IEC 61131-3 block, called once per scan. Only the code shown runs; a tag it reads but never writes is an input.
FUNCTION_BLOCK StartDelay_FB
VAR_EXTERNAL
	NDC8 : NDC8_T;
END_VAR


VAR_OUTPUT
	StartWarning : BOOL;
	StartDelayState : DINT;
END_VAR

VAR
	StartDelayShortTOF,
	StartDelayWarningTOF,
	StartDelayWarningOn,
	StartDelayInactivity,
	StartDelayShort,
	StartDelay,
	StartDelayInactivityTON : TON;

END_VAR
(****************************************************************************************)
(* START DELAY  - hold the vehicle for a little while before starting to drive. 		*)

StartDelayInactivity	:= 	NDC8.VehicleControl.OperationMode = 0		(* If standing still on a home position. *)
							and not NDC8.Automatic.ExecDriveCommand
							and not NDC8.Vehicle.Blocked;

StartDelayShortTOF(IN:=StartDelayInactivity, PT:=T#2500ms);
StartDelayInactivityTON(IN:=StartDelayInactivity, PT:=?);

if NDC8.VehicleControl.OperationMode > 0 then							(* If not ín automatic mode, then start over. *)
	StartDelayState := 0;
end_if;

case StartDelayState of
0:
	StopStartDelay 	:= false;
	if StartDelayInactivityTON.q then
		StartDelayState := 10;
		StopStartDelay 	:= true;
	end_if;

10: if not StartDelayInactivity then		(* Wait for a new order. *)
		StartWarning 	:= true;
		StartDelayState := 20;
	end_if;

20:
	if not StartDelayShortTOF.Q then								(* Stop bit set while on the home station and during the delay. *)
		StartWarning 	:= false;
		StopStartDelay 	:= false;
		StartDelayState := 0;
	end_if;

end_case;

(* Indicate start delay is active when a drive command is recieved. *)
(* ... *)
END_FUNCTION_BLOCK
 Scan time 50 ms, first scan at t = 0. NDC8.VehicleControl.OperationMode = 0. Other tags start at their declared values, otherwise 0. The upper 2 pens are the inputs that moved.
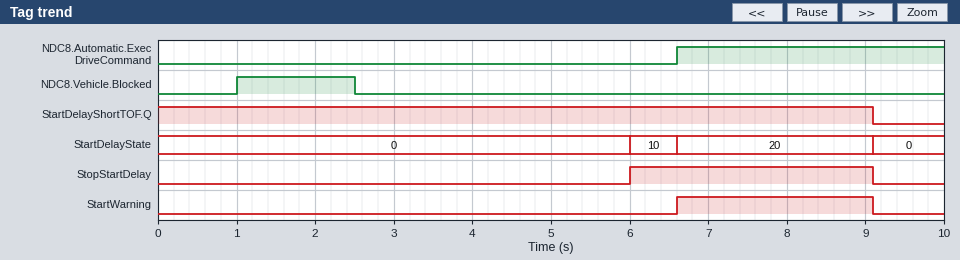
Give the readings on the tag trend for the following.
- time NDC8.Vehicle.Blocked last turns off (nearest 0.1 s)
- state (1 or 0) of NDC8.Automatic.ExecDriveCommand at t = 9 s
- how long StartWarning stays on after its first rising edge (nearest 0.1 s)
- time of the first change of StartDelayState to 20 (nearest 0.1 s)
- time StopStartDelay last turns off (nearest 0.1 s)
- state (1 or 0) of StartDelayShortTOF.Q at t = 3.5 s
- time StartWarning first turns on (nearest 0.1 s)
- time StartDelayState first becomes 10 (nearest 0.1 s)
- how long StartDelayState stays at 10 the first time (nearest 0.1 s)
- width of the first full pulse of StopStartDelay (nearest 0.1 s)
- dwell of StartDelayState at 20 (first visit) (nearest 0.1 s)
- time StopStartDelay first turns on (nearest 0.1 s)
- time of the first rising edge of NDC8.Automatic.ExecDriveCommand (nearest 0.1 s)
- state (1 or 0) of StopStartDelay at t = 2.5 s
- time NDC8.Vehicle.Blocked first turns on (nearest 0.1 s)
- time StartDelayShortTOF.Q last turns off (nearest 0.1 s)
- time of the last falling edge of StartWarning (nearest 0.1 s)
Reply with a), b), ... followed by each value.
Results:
a) 2.5 s
b) 1
c) 2.5 s
d) 6.6 s
e) 9.1 s
f) 1
g) 6.6 s
h) 6.0 s
i) 0.6 s
j) 3.1 s
k) 2.5 s
l) 6.0 s
m) 6.6 s
n) 0
o) 1.0 s
p) 9.1 s
q) 9.1 s
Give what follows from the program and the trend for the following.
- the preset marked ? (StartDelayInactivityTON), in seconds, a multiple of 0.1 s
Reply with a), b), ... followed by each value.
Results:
a) 3.5 s
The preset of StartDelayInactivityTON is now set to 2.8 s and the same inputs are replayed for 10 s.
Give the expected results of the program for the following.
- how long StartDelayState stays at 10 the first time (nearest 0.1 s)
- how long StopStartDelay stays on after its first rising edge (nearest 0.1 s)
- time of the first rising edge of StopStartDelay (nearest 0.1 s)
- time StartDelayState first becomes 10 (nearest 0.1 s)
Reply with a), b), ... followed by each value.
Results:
a) 1.3 s
b) 3.8 s
c) 5.3 s
d) 5.3 s
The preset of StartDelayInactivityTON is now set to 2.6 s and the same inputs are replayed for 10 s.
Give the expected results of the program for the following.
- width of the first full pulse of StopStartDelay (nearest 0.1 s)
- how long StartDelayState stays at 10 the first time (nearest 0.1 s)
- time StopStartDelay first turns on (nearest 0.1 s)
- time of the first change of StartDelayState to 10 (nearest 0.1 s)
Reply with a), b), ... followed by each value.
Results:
a) 4.0 s
b) 1.5 s
c) 5.1 s
d) 5.1 s
